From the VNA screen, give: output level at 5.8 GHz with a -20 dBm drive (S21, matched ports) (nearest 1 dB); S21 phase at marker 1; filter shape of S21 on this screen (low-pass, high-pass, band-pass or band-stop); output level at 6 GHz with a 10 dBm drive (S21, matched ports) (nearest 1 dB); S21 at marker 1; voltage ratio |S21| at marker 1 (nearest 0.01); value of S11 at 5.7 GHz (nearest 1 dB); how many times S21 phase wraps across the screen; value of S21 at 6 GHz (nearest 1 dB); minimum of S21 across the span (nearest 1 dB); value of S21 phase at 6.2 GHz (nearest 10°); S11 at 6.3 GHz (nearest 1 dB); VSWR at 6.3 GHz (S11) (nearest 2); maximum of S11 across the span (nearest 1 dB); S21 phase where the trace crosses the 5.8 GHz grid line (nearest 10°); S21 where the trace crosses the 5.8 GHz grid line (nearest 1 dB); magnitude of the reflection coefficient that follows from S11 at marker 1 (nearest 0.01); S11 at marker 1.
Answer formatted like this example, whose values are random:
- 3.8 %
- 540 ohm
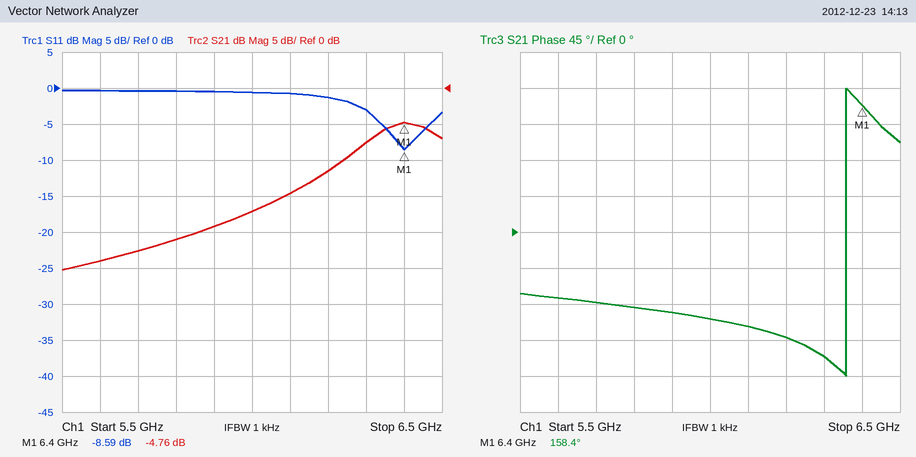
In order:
- -41 dBm
- 158.4°
- high-pass
- -7 dBm
- -4.76 dB
- 0.58
- 0 dB
- 1
- -17 dB
- -25 dB
- -130°
- -3 dB
- 6
- 0 dB
- -90°
- -21 dB
- 0.37
- -8.59 dB
